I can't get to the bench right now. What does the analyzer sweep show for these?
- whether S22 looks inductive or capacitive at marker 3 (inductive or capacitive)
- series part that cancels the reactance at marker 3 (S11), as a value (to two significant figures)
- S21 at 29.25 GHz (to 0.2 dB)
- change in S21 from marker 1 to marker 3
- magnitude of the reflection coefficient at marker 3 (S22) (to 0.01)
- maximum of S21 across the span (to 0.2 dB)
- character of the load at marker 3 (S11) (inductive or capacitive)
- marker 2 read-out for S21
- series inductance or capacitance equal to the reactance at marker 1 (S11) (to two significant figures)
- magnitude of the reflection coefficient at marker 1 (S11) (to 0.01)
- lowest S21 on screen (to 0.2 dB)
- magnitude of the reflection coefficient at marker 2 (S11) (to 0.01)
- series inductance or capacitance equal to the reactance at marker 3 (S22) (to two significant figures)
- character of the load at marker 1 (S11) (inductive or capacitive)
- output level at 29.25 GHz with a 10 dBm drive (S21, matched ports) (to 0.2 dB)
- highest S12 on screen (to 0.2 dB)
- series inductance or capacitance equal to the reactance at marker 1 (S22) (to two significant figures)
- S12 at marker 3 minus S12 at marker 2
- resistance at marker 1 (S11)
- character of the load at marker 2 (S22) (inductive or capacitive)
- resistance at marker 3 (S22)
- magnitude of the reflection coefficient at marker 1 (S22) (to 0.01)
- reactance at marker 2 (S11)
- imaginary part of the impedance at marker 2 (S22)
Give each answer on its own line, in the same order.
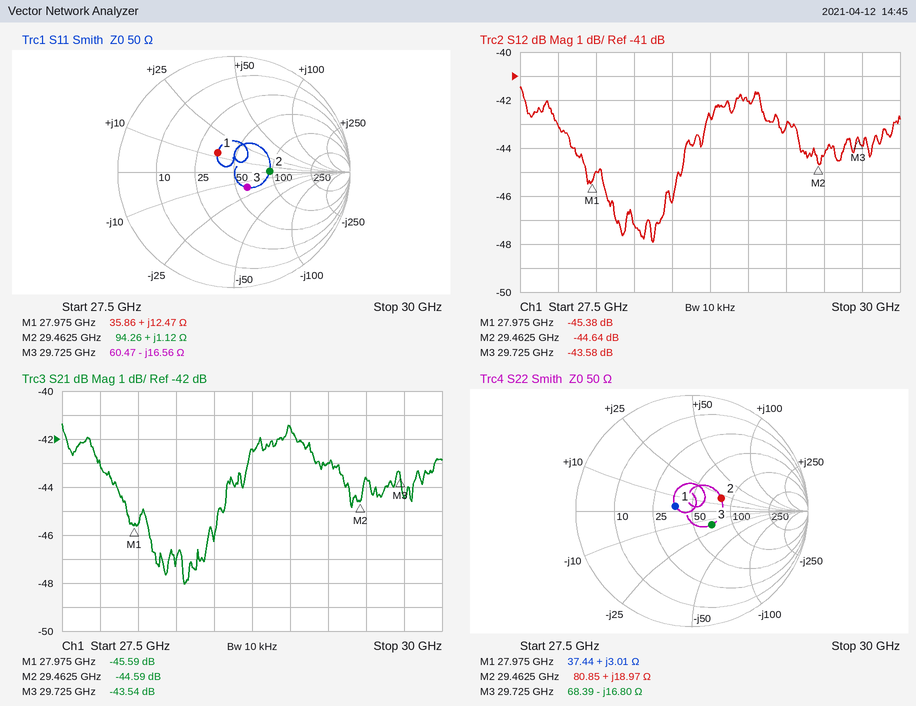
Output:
capacitive
89 pH
-43.0 dB
2.05 dB
0.21
-41.4 dB
capacitive
-44.59 dB
71 pH
0.22
-48.0 dB
0.31
320 fF
inductive
-33.0 dBm
-41.4 dB
17 pH
1.06 dB
35.86 Ω
inductive
68.39 Ω
0.15
+1.12 Ω
+18.97 Ω
